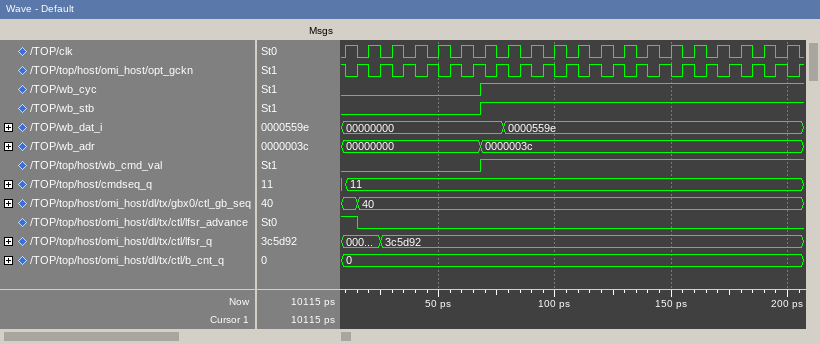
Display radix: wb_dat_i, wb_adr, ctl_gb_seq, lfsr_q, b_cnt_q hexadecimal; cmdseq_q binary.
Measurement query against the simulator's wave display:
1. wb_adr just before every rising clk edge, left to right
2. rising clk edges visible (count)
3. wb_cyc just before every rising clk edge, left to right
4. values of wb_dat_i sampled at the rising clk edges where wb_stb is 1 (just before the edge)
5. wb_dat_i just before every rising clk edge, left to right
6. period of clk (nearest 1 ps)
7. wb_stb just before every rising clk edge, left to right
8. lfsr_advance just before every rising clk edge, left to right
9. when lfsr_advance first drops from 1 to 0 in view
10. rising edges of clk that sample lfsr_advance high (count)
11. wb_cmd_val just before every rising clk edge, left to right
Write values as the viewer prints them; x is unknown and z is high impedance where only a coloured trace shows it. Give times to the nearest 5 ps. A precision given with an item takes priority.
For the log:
00000000, 00000000, 00000000, 00000000, 00000000, 00000000, 0000003c, 0000003c, 0000003c, 0000003c, 0000003c, 0000003c, 0000003c, 0000003c, 0000003c, 0000003c, 0000003c, 0000003c, 0000003c, 0000003c
20
0 0 0 0 0 0 1 1 1 1 1 1 1 1 1 1 1 1 1 1
00000000, 0000559e, 0000559e, 0000559e, 0000559e, 0000559e, 0000559e, 0000559e, 0000559e, 0000559e, 0000559e, 0000559e, 0000559e, 0000559e
00000000, 00000000, 00000000, 00000000, 00000000, 00000000, 00000000, 0000559e, 0000559e, 0000559e, 0000559e, 0000559e, 0000559e, 0000559e, 0000559e, 0000559e, 0000559e, 0000559e, 0000559e, 0000559e
10 ps
0 0 0 0 0 0 1 1 1 1 1 1 1 1 1 1 1 1 1 1
1 0 0 0 0 0 0 0 0 0 0 0 0 0 0 0 0 0 0 0
15 ps
1
0 0 0 0 0 0 1 1 1 1 1 1 1 1 1 1 1 1 1 1
